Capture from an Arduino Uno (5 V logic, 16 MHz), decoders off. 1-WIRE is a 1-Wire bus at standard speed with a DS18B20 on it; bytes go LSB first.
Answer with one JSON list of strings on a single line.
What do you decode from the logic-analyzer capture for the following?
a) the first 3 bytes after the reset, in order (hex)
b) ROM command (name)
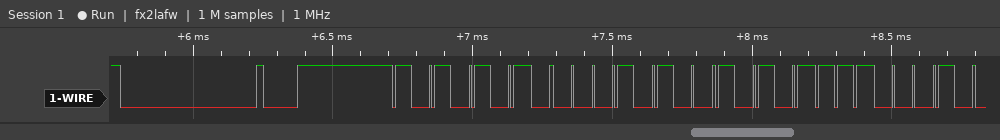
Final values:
["55 28 F5", "Match ROM"]
